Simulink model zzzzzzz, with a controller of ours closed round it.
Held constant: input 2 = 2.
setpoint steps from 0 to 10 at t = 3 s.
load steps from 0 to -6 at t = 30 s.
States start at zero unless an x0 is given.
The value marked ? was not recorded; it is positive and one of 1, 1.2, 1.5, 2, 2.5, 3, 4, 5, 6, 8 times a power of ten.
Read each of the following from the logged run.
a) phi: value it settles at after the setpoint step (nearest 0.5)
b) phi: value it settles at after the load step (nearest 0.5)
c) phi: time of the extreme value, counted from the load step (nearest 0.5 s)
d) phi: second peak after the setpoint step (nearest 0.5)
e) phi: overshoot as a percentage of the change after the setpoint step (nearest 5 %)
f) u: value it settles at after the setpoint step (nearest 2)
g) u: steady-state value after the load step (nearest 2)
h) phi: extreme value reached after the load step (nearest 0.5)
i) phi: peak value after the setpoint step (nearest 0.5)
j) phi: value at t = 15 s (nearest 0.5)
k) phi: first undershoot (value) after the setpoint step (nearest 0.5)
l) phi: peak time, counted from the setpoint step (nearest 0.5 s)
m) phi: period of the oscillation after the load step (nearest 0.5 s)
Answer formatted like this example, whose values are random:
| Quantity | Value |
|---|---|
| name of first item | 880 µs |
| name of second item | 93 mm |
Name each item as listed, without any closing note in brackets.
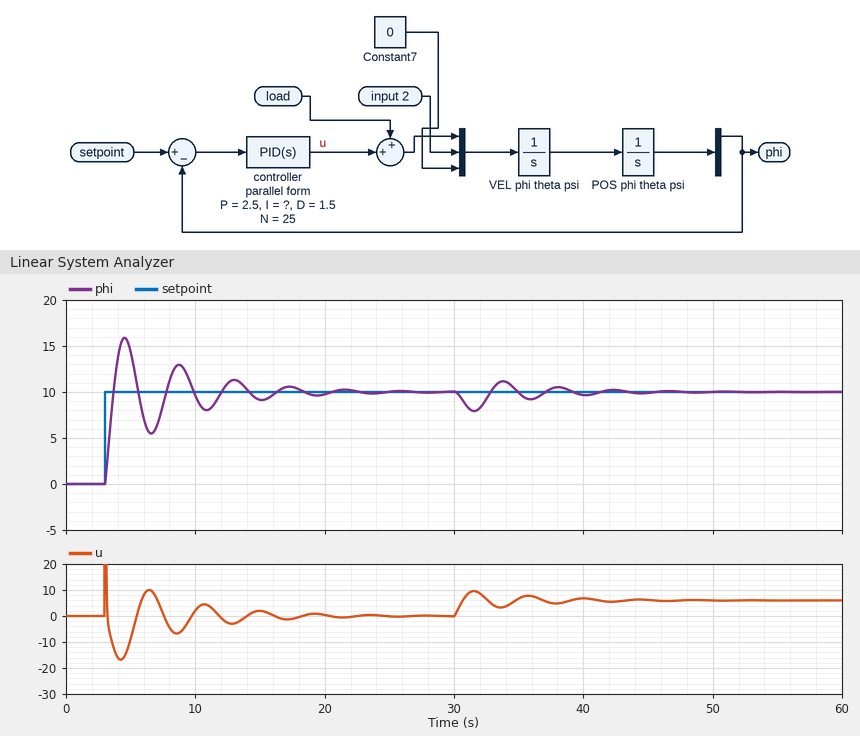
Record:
| Quantity | Value |
|---|---|
| phi: value it settles at after the setpoint step | 10.0 |
| phi: value it settles at after the load step | 10.0 |
| phi: time of the extreme value, counted from the load step | 1.5 s |
| phi: second peak after the setpoint step | 13.0 |
| phi: overshoot as a percentage of the change after the setpoint step | 60 % |
| u: value it settles at after the setpoint step | 0 |
| u: steady-state value after the load step | 6 |
| phi: extreme value reached after the load step | 8.0 |
| phi: peak value after the setpoint step | 16.0 |
| phi: value at t = 15 s | 9.0 |
| phi: first undershoot (value) after the setpoint step | 5.5 |
| phi: peak time, counted from the setpoint step | 1.5 s |
| phi: period of the oscillation after the load step | 4.5 s |
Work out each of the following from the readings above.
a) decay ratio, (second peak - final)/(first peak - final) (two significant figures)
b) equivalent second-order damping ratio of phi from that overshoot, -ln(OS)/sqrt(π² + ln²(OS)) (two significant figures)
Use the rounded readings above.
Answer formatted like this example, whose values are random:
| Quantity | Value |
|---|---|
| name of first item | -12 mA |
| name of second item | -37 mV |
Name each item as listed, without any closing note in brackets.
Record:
| Quantity | Value |
|---|---|
| decay ratio, (second peak - final)/(first peak - final) | 0.50 |
| equivalent second-order damping ratio of phi from that overshoot, -ln(OS)/sqrt(π² + ln²(OS)) | 0.16 |
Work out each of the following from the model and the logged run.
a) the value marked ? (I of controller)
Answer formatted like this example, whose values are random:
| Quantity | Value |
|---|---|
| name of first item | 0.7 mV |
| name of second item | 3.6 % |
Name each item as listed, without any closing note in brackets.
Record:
| Quantity | Value |
|---|---|
| the value marked ? | 2.5 |
